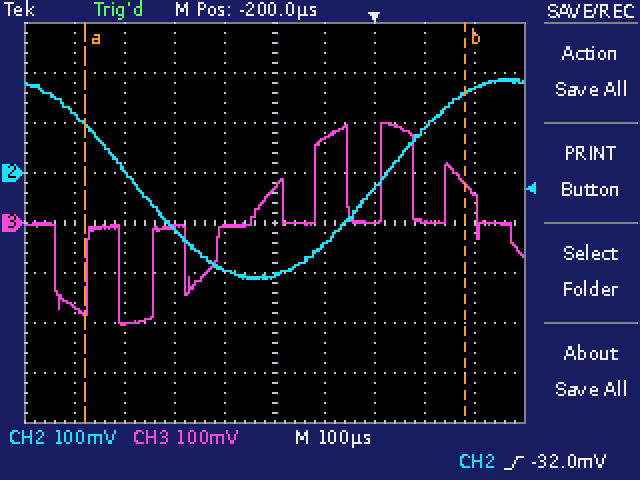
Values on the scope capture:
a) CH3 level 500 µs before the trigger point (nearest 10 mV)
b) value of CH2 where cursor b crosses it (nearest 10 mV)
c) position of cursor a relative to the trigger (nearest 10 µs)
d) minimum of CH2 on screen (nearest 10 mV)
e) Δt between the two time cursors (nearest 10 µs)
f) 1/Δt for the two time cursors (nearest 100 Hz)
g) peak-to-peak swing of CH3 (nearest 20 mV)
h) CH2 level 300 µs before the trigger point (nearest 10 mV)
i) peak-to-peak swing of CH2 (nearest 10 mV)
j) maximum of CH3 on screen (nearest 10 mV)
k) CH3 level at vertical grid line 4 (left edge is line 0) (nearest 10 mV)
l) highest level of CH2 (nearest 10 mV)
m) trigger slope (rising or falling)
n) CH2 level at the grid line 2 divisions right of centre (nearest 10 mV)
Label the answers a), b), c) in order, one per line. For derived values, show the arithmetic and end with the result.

a) -200 mV
b) 160 mV
c) -580 µs
d) -210 mV
e) 760 µs
f) 1 / 760 µs ≈ 1.3 kHz
g) 400 mV
h) -190 mV
i) 190 mV − (-210 mV) = 400 mV
j) 200 mV
k) -10 mV
l) 190 mV
m) rising
n) -30 mV
